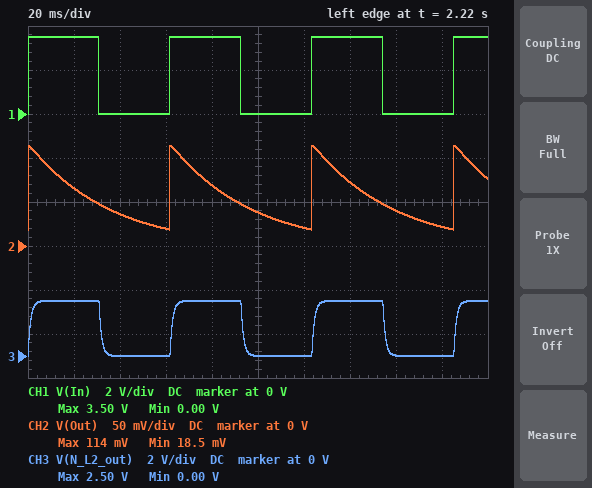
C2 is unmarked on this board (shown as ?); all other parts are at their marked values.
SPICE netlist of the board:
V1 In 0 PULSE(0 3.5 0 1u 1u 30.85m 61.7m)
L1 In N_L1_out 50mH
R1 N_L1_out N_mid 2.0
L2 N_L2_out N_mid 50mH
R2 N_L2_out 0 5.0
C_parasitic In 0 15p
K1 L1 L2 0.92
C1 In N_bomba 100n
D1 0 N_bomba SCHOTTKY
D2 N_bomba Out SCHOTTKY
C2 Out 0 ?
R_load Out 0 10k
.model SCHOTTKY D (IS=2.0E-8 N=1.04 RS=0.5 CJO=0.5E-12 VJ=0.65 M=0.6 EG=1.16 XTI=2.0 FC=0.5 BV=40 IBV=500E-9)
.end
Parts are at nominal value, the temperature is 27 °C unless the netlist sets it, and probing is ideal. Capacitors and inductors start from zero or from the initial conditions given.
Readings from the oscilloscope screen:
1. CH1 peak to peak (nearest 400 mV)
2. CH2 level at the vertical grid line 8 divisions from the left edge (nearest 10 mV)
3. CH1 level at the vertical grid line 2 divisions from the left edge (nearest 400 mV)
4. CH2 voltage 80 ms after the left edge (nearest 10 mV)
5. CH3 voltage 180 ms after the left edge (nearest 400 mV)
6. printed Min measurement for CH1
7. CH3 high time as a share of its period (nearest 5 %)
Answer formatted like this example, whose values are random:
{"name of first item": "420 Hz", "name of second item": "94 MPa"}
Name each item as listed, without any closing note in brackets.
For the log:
{"CH1 peak to peak": "3.6 V", "CH2 level at the vertical grid line 8 divisions from the left edge": "40 mV", "CH1 level at the vertical grid line 2 divisions from the left edge": "0 V", "CH2 voltage 80 ms after the left edge": "70 mV", "CH3 voltage 180 ms after the left edge": "0 V", "printed Min measurement for CH1": "0.00 V", "CH3 high time as a share of its period": "50 %"}
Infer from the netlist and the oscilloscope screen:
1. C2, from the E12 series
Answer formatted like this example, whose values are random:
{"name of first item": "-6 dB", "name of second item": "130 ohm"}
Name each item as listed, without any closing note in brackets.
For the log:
{"C2, from the E12 series": "3.3 µF"}
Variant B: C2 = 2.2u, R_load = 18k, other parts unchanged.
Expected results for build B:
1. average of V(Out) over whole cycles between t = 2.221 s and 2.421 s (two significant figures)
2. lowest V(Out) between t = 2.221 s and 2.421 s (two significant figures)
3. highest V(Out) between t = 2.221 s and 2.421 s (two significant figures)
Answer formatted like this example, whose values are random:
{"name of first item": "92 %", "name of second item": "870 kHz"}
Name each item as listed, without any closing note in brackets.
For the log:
{"average of V(Out) over whole cycles between t = 2.221 s and 2.421 s": "96 mV", "lowest V(Out) between t = 2.221 s and 2.421 s": "40 mV", "highest V(Out) between t = 2.221 s and 2.421 s": "180 mV"}
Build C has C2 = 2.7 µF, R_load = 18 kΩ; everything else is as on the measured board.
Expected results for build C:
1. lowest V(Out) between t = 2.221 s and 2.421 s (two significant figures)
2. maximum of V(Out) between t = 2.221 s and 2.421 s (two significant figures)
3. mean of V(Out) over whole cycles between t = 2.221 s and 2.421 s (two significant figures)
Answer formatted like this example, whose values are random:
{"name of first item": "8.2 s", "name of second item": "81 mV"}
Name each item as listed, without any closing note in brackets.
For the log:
{"lowest V(Out) between t = 2.221 s and 2.421 s": "48 mV", "maximum of V(Out) between t = 2.221 s and 2.421 s": "160 mV", "mean of V(Out) over whole cycles between t = 2.221 s and 2.421 s": "96 mV"}
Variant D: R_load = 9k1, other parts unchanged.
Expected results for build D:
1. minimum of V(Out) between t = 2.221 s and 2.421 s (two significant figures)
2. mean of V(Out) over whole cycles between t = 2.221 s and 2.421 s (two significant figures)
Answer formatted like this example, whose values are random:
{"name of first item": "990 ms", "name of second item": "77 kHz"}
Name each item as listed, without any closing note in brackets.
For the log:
{"minimum of V(Out) between t = 2.221 s and 2.421 s": "15 mV", "mean of V(Out) over whole cycles between t = 2.221 s and 2.421 s": "49 mV"}
